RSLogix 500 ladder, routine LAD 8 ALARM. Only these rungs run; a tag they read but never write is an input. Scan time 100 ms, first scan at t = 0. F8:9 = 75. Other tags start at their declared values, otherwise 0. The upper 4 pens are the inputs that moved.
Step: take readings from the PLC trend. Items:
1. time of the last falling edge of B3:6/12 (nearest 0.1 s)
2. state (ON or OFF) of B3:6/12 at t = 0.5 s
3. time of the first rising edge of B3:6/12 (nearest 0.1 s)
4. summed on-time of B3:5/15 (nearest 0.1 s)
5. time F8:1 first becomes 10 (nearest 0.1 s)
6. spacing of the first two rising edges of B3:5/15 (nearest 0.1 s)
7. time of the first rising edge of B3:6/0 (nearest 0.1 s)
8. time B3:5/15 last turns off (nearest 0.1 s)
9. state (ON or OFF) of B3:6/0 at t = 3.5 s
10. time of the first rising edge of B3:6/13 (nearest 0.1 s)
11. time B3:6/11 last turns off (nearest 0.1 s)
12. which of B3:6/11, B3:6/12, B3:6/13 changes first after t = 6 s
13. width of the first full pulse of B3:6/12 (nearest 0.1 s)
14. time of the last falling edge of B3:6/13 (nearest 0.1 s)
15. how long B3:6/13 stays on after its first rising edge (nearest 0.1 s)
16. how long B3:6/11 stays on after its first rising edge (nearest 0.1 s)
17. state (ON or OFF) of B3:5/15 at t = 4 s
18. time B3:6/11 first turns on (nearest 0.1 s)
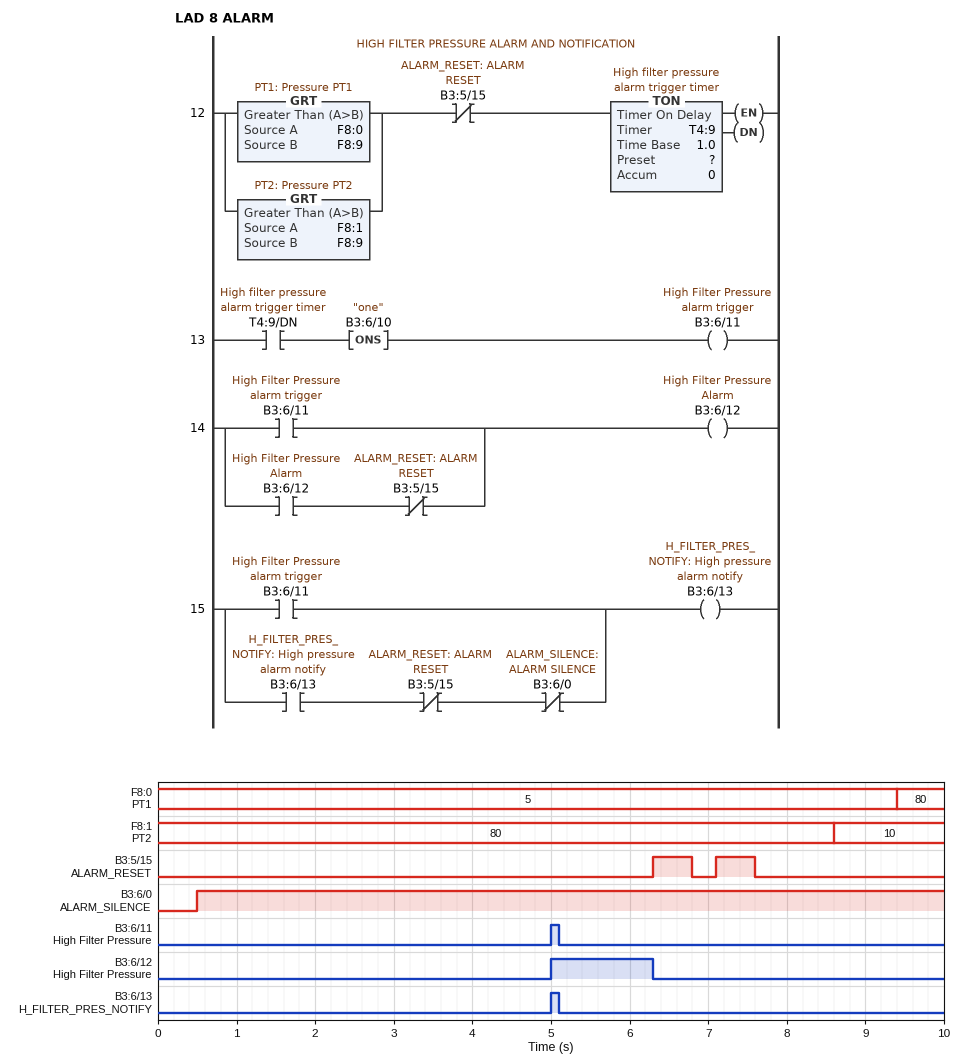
6.3 s
OFF
5.0 s
1.0 s
8.6 s
0.8 s
0.5 s
7.6 s
ON
5.0 s
5.1 s
B3:6/12
1.3 s
5.1 s
0.1 s
0.1 s
OFF
5.0 s
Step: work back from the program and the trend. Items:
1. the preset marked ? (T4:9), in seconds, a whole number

5 s
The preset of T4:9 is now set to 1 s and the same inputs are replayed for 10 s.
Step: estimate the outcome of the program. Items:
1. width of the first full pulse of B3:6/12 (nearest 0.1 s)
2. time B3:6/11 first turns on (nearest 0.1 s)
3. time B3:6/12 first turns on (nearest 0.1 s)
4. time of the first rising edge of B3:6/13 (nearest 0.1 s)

5.3 s
1.0 s
1.0 s
1.0 s
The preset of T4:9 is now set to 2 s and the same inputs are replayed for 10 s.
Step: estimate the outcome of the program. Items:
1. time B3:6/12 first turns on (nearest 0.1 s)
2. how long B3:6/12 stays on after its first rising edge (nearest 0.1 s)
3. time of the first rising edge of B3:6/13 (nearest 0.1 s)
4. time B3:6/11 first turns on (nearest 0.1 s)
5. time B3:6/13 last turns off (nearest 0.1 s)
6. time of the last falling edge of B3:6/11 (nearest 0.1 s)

2.0 s
4.3 s
2.0 s
2.0 s
2.1 s
2.1 s
